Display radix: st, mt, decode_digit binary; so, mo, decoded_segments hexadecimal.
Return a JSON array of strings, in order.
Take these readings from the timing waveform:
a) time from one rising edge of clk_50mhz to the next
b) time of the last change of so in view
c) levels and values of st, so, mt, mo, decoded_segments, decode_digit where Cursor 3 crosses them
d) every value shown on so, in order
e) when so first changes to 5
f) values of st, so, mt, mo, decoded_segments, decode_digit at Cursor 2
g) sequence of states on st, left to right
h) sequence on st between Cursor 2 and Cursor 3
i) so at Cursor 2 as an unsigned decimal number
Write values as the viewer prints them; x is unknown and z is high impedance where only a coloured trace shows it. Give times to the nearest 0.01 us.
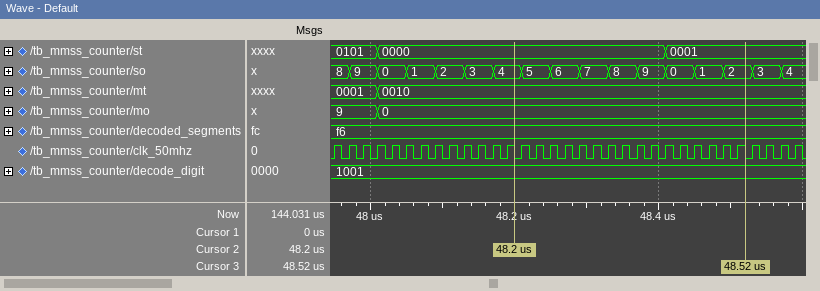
["0.02 us", "48.57 us", "st=0001, so=2, mt=0010, mo=0, decoded_segments=f6, decode_digit=1001", "8, 9, 0, 1, 2, 3, 4, 5, 6, 7, 8, 9, 0, 1, 2, 3, 4", "48.21 us", "st=0000, so=4, mt=0010, mo=0, decoded_segments=f6, decode_digit=1001", "0101, 0000, 0001", "0000, 0001", "4"]
